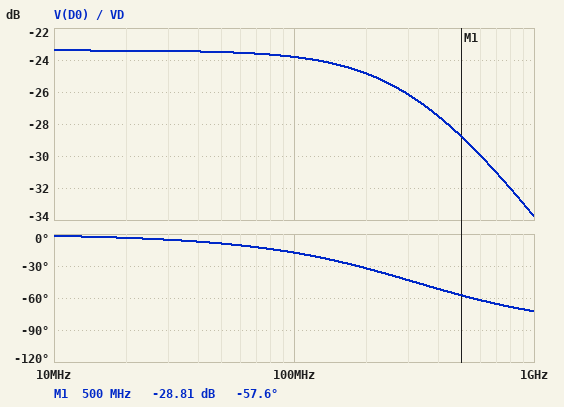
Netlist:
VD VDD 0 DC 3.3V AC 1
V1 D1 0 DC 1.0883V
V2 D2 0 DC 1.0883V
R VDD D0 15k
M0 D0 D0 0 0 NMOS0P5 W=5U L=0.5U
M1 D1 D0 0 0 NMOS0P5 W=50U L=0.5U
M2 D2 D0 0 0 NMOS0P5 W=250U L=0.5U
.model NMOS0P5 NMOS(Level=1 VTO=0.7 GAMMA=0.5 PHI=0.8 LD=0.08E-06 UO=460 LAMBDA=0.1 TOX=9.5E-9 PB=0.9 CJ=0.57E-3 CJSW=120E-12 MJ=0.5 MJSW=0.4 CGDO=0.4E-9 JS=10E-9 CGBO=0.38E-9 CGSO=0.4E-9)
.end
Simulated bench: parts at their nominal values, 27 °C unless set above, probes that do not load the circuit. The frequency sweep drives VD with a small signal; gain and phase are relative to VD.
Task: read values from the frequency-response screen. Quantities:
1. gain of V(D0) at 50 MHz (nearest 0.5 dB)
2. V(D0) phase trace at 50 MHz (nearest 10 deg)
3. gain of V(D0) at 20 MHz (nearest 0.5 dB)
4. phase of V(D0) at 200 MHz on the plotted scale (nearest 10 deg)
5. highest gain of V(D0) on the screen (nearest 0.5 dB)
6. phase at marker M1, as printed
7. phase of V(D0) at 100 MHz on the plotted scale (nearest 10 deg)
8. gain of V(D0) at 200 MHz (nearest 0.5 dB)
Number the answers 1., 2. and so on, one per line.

1. -23.5 dB
2. -10 deg
3. -23.5 dB
4. -30 deg
5. -23.5 dB
6. -57.6 deg
7. -20 deg
8. -25.0 dB
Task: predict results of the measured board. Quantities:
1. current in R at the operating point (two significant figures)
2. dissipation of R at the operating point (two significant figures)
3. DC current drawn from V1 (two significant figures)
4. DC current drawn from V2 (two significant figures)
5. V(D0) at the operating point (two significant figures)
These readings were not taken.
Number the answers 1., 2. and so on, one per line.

1. 150 µA
2. 340 µW
3. 1.5 mA
4. 7.6 mA
5. 1.0 V
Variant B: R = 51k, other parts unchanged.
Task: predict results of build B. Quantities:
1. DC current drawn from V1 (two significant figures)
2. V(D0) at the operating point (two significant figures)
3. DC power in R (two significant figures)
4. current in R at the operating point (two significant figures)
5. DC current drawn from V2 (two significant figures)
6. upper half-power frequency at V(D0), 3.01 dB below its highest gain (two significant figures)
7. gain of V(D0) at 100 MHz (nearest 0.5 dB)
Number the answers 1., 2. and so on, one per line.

1. 480 µA
2. 890 mV
3. 110 µW
4. 47 µA
5. 2.4 mA
6. 170 MHz
7. -30.0 dB
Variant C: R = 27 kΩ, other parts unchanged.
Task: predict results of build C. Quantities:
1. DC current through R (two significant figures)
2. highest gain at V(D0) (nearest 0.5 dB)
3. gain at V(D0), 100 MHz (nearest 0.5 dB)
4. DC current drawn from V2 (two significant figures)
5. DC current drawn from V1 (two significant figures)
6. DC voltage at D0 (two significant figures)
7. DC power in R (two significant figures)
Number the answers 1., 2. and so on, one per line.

1. 87 µA
2. -26.0 dB
3. -26.5 dB
4. 4.4 mA
5. 880 µA
6. 950 mV
7. 200 µW
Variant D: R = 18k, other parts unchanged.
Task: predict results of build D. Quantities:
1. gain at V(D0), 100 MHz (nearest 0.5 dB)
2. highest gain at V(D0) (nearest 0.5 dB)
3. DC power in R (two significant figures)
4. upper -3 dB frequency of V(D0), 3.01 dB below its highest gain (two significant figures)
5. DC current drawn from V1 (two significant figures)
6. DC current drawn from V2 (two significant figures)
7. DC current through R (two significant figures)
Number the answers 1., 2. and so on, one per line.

1. -24.5 dB
2. -24.0 dB
3. 290 µW
4. 290 MHz
5. 1.3 mA
6. 6.4 mA
7. 130 µA
